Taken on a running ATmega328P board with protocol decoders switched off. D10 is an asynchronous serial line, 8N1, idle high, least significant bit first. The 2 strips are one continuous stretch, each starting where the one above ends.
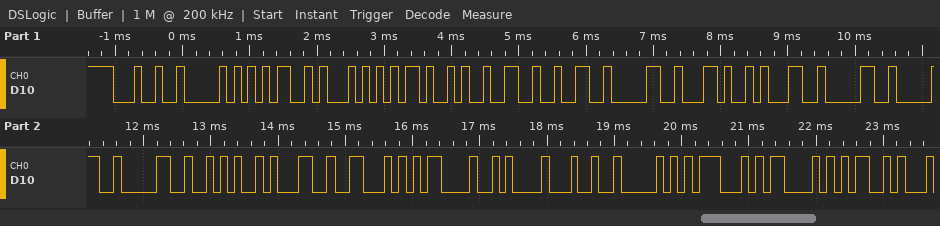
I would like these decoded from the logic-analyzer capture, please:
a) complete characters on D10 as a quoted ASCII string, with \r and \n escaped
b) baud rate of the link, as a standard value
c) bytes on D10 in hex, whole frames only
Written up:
"$PMTK220,1000*1F\r\n$PGCM"
9600 baud
24 50 4D 54 4B 32 32 30 2C 31 30 30 30 2A 31 46 0D 0A 24 50 47 43 4D
